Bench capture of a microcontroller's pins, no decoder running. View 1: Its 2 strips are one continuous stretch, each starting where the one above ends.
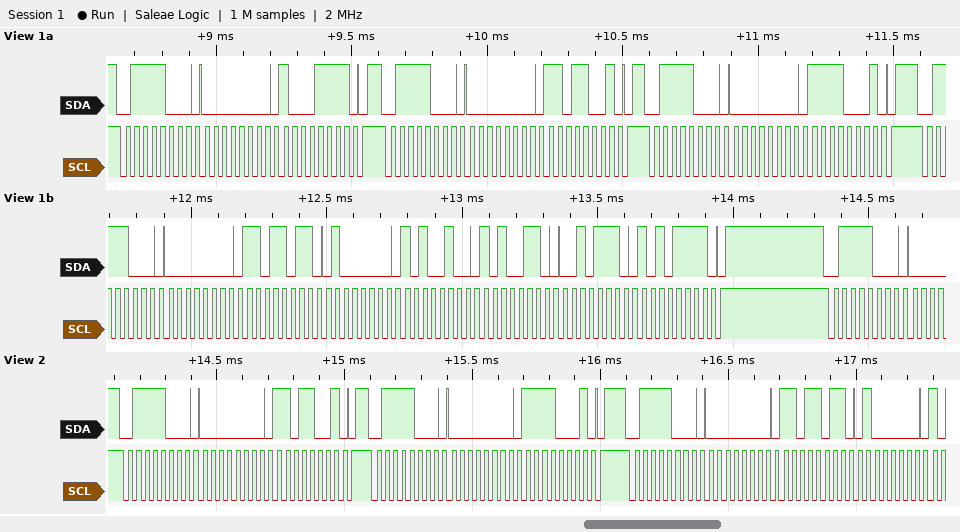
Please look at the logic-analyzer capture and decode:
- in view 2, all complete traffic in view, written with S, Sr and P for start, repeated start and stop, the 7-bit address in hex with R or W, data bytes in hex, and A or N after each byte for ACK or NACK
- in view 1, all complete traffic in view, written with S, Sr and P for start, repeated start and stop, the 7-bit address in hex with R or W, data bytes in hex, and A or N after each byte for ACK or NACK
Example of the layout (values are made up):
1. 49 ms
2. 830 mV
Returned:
1. S 3CW A 00 A D9 A P S 3CW A 00 A F1 A P S 3CW A 00 A DB A 40 A
2. S 3CW A 00 A 8F A P S 3CW A 00 A D9 A P S 3CW A 00 A F1 A P S 3CW A 00 A DB A 40 A A4 A A6 A 2E A AF A P S 3CW A
